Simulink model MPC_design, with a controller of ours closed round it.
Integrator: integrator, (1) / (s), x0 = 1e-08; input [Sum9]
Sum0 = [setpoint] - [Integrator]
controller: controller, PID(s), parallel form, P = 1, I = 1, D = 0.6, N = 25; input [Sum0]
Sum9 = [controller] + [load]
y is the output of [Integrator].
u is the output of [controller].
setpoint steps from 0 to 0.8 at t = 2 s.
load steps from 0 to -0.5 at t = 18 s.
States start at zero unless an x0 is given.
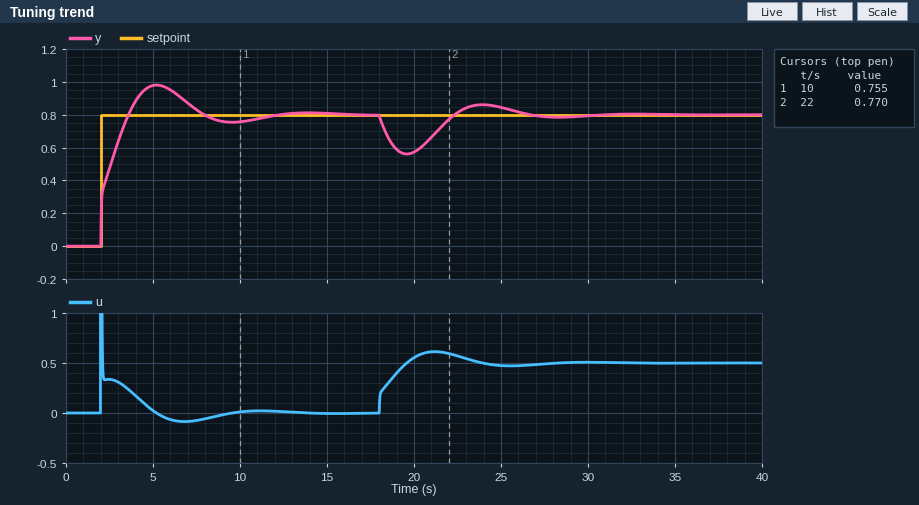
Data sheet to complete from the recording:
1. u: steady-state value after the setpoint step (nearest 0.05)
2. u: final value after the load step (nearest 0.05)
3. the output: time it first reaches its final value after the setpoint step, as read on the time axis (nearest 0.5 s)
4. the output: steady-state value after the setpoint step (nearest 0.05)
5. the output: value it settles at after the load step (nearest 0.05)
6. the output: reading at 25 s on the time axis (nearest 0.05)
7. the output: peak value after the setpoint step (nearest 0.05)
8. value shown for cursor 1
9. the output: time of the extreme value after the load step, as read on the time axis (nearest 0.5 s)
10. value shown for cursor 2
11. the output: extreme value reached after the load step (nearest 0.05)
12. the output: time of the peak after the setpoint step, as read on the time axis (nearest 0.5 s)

0.00
0.50
3.5 s
0.80
0.80
0.85
1.00
0.755
19.5 s
0.770
0.55
5.0 s
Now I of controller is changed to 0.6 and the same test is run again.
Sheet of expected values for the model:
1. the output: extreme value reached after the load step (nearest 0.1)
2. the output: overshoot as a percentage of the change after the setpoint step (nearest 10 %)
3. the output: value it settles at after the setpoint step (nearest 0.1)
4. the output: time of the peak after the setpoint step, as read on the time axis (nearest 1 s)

0.5
20 %
0.8
6 s
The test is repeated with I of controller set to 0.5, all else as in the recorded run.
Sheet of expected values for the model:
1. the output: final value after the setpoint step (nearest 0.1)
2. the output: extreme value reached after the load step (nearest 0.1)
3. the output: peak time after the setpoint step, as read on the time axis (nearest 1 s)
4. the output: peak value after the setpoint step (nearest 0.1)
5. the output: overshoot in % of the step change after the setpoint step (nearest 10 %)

0.8
0.5
6 s
0.9
20 %
